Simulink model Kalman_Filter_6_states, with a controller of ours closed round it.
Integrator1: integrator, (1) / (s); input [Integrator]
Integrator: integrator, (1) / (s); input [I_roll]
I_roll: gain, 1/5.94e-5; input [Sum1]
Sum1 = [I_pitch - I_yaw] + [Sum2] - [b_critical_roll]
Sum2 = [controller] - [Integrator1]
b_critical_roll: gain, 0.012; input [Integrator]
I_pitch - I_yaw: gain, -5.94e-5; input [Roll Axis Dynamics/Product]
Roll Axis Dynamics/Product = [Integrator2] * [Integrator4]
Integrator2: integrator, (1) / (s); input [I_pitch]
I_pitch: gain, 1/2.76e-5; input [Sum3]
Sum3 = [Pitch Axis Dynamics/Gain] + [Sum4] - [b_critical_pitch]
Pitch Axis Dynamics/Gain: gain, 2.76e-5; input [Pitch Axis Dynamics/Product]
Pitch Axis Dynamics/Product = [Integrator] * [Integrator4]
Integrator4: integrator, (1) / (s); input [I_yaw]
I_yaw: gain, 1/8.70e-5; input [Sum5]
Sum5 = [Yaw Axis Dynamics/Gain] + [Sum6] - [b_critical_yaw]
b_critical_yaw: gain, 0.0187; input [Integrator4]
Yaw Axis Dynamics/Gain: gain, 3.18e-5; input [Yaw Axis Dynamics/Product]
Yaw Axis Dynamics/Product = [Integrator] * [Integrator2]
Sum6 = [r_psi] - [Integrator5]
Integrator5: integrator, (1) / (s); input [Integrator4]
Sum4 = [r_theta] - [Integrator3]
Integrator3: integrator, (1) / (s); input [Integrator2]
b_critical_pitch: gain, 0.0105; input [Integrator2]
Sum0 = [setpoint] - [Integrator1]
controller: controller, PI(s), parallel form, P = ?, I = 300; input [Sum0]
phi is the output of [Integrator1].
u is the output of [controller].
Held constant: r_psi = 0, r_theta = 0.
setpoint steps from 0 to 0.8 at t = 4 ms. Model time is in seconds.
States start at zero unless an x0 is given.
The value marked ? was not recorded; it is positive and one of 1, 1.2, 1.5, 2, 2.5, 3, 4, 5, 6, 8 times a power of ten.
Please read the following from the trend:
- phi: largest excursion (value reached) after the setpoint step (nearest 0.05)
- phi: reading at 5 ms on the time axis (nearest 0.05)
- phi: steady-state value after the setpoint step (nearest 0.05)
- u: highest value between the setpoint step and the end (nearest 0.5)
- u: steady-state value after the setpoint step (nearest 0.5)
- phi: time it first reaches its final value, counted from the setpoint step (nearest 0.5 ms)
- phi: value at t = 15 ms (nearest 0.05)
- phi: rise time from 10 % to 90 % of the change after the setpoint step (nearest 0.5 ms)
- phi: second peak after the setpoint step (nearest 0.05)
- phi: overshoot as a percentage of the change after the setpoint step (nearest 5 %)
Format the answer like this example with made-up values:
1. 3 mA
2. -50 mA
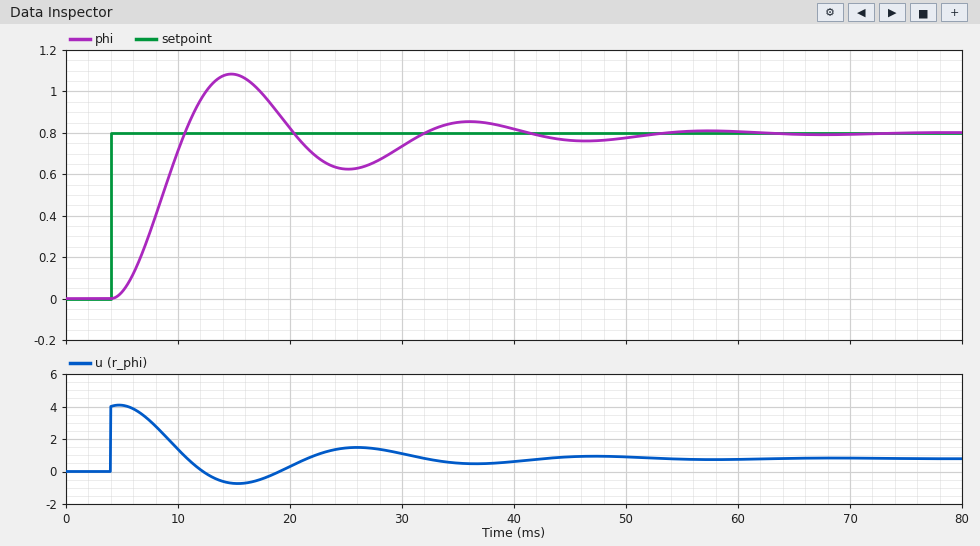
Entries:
1. 1.10
2. 0.05
3. 0.80
4. 4.0
5. 1.0
6. 6.5 ms
7. 1.10
8. 4.5 ms
9. 0.85
10. 35 %
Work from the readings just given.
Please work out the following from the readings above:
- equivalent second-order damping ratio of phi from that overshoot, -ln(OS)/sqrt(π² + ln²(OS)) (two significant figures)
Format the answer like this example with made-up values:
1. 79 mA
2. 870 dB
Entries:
1. 0.32
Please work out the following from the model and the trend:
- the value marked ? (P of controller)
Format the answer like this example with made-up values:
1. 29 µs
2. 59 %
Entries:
1. 5
